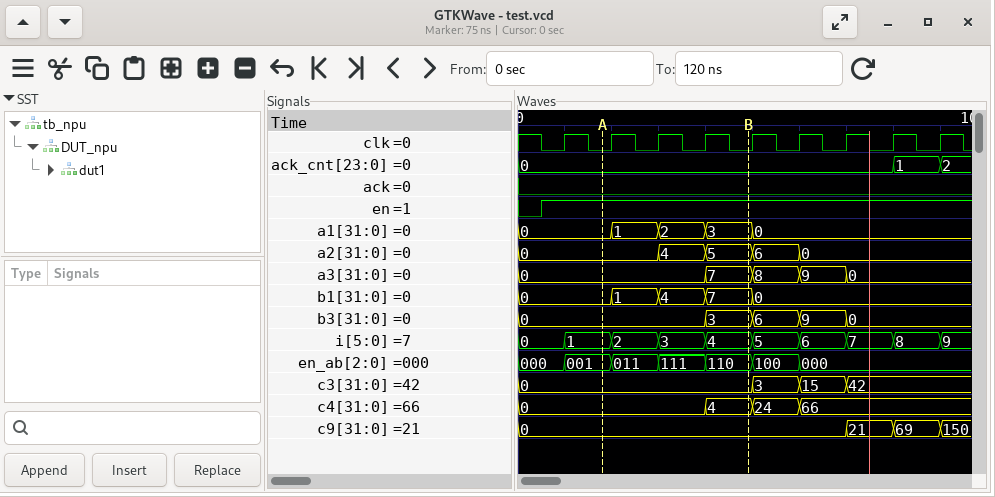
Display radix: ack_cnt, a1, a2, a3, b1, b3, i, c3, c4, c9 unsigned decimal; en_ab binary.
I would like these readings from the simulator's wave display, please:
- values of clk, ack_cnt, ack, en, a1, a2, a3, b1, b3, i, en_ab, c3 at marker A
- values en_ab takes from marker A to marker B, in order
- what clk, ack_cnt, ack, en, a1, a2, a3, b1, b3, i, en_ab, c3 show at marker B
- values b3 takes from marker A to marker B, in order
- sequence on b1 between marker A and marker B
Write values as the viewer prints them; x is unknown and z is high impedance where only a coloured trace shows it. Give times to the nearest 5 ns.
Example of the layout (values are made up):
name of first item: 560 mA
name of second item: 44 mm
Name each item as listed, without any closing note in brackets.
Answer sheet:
values of clk, ack_cnt, ack, en, a1, a2, a3, b1, b3, i, en_ab, c3 at marker A: clk=0, ack_cnt=0, ack=0, en=1, a1=0, a2=0, a3=0, b1=0, b3=0, i=1, en_ab=001, c3=0
values en_ab takes from marker A to marker B, in order: 001, 011, 111, 110
what clk, ack_cnt, ack, en, a1, a2, a3, b1, b3, i, en_ab, c3 show at marker B: clk=0, ack_cnt=0, ack=0, en=1, a1=3, a2=5, a3=7, b1=7, b3=3, i=4, en_ab=110, c3=0
values b3 takes from marker A to marker B, in order: 0, 3
sequence on b1 between marker A and marker B: 0, 1, 4, 7
